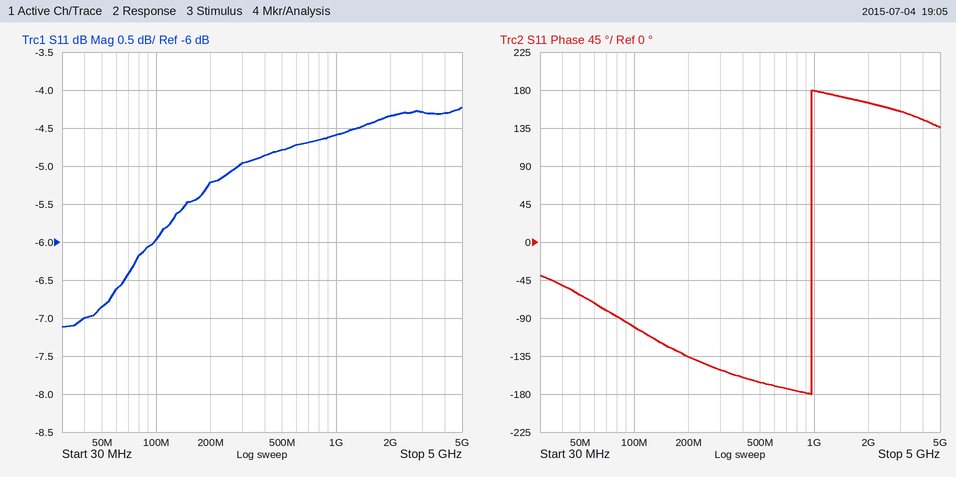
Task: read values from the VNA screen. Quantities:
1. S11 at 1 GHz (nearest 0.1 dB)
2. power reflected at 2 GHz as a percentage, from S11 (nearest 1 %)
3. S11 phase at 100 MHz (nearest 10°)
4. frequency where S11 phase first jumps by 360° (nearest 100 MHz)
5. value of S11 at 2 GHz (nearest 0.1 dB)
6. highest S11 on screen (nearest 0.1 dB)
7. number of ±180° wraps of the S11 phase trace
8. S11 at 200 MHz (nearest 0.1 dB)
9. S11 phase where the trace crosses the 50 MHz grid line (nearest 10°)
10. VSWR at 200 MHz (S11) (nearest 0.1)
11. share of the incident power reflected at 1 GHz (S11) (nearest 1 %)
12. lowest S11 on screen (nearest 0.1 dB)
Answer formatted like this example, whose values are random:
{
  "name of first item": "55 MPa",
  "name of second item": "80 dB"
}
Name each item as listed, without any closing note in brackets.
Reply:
{
  "S11 at 1 GHz": "-4.6 dB",
  "power reflected at 2 GHz as a percentage, from S11": "37 %",
  "S11 phase at 100 MHz": "-100°",
  "frequency where S11 phase first jumps by 360°": "1.0 GHz",
  "value of S11 at 2 GHz": "-4.3 dB",
  "highest S11 on screen": "-4.2 dB",
  "number of ±180° wraps of the S11 phase trace": "1",
  "S11 at 200 MHz": "-5.2 dB",
  "S11 phase where the trace crosses the 50 MHz grid line": "-60°",
  "VSWR at 200 MHz (S11)": "3.4",
  "share of the incident power reflected at 1 GHz (S11)": "35 %",
  "lowest S11 on screen": "-7.1 dB"
}
